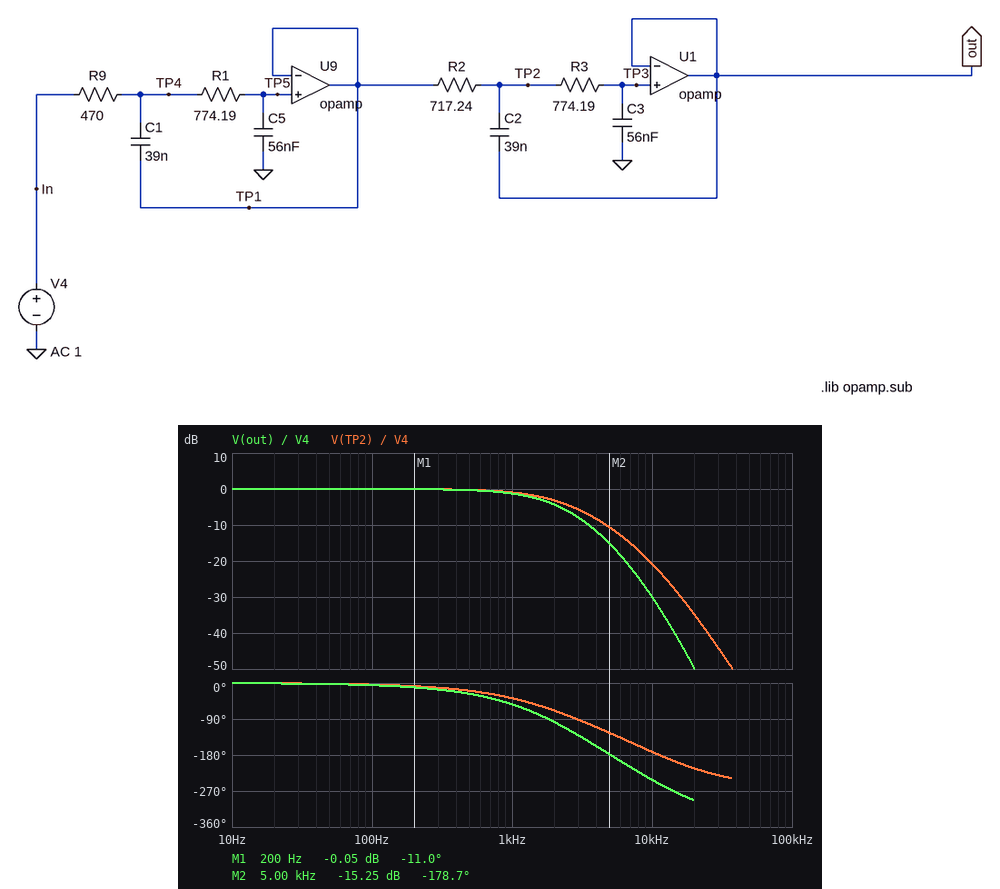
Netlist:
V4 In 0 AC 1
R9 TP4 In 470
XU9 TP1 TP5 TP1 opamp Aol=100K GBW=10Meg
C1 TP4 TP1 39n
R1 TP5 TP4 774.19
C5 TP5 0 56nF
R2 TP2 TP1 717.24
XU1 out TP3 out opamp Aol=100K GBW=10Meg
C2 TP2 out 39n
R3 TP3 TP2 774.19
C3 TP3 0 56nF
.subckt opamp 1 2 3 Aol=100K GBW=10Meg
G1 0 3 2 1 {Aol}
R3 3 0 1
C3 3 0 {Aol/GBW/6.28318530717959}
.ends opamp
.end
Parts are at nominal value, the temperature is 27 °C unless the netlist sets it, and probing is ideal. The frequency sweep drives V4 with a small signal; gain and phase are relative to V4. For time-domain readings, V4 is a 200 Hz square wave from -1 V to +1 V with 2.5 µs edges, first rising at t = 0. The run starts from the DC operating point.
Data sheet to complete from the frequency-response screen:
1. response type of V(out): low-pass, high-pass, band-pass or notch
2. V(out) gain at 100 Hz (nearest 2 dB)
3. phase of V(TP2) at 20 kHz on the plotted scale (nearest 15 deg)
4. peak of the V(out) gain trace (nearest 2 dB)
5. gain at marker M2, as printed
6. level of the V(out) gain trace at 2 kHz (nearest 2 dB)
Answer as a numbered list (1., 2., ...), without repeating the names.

1. low-pass
2. 0 dB
3. -210 deg
4. 0 dB
5. -15.25 dB
6. -4 dB
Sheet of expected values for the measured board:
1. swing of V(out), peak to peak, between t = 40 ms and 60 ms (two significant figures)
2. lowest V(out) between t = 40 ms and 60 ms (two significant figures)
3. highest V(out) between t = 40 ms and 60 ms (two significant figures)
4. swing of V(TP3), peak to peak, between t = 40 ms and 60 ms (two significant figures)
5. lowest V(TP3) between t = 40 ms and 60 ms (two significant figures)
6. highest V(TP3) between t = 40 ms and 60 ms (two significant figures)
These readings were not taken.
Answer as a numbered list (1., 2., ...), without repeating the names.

1. 2.0 V
2. -1.0 V
3. 1.0 V
4. 2.0 V
5. -1.0 V
6. 1.0 V
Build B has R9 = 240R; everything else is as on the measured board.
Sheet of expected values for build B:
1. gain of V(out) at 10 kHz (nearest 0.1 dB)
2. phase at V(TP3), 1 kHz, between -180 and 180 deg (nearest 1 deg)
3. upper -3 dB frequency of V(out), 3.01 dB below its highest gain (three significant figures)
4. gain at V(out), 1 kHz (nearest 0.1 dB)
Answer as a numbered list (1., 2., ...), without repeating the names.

1. -27.4 dB
2. -49 deg
3. 1.73 kHz
4. -1.1 dB
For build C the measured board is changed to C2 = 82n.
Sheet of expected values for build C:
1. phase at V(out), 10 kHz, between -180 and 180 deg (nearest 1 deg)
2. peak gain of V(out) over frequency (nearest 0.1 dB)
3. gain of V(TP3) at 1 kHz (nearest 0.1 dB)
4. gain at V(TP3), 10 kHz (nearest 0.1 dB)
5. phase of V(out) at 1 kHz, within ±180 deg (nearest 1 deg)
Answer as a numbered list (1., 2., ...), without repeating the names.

1. 94 deg
2. 0 dB
3. -0.9 dB
4. -34.2 dB
5. -55 deg
